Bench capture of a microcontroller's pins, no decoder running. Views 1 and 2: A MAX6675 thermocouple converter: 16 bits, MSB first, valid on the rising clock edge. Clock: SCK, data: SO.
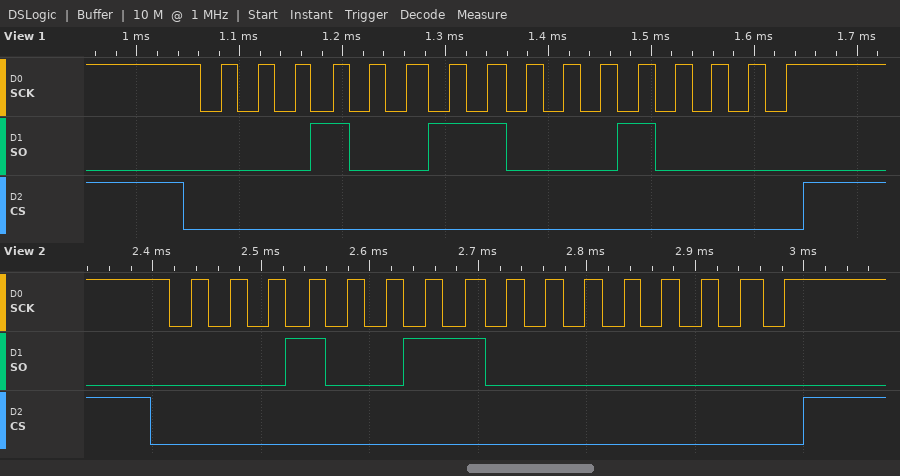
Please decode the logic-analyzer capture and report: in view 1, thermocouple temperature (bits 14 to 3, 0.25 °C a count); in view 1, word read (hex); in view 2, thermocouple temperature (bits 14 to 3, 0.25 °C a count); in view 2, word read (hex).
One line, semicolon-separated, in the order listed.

152.50 °C; 0x1310; 152.00 °C; 0x1300
